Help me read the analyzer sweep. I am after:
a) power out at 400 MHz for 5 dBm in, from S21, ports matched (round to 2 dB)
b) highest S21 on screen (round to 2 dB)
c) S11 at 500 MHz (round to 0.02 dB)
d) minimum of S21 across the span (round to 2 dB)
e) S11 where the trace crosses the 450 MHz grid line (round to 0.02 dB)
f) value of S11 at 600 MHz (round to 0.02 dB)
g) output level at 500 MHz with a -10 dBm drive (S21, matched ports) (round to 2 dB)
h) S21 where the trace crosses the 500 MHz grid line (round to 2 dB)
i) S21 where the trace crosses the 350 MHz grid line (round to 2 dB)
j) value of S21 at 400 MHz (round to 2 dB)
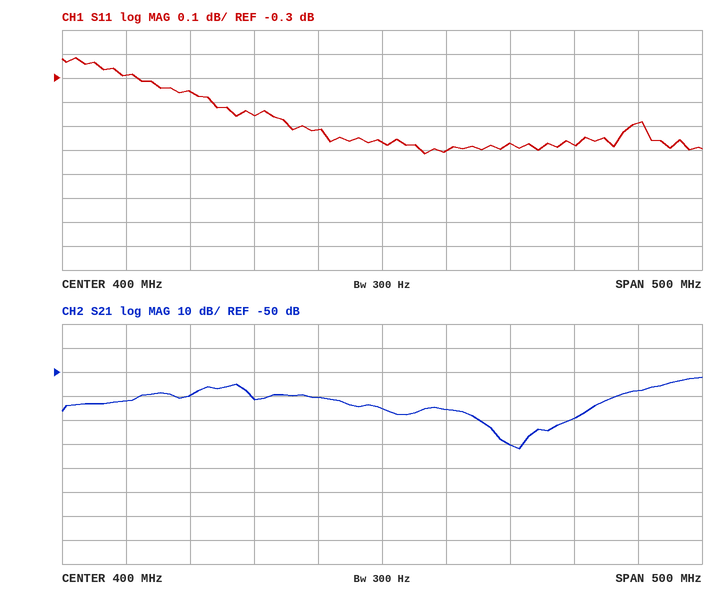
-60 dBm
-52 dB
-0.58 dB
-82 dB
-0.60 dB
-0.48 dB
-90 dBm
-80 dB
-60 dB
-66 dB
